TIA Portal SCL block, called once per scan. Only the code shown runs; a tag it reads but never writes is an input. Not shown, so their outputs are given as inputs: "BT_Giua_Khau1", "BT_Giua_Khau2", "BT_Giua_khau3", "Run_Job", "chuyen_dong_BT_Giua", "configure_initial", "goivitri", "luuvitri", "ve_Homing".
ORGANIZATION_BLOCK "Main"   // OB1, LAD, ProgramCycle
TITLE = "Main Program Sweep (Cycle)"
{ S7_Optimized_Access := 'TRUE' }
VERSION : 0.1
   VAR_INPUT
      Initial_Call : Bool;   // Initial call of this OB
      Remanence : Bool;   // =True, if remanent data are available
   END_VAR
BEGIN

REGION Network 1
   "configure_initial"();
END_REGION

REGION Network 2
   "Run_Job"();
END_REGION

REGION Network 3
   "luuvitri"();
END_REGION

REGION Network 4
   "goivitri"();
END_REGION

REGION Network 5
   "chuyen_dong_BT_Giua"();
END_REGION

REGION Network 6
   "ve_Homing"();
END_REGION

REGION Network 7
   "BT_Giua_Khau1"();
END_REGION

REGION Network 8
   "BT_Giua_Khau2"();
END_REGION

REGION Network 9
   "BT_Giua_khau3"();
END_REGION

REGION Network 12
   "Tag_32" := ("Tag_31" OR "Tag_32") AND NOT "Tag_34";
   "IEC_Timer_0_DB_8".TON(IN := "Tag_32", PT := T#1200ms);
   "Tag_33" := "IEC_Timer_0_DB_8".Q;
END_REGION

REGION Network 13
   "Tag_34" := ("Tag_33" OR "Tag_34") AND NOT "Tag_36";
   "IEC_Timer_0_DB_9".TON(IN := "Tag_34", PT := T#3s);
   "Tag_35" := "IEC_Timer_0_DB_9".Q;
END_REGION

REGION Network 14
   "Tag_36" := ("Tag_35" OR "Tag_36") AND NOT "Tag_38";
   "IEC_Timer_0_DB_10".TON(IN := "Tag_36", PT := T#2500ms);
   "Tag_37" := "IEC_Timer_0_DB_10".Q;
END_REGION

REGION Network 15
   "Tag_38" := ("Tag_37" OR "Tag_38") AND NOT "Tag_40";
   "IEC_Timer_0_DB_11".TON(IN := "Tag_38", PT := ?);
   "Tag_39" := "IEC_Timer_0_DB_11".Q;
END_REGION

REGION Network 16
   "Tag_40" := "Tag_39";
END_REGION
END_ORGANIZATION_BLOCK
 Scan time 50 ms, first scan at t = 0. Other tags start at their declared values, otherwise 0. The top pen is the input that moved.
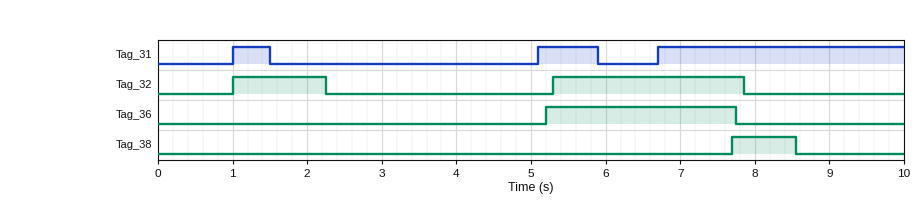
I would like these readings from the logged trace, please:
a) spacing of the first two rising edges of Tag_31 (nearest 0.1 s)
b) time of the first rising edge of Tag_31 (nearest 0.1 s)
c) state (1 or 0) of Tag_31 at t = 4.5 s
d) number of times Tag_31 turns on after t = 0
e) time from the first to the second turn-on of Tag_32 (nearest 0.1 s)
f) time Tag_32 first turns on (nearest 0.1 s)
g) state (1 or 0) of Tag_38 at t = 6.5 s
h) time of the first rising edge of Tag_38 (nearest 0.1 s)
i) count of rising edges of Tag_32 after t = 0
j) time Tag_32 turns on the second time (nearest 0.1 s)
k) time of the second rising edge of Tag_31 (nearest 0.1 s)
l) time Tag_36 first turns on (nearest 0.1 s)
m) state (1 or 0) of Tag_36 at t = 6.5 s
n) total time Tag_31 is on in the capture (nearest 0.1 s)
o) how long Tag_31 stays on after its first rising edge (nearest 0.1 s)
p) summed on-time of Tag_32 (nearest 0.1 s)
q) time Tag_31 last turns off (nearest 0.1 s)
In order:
4.1 s
1.0 s
0
3
4.3 s
1.0 s
0
7.7 s
2
5.3 s
5.1 s
5.2 s
1
4.6 s
0.5 s
3.8 s
5.9 s
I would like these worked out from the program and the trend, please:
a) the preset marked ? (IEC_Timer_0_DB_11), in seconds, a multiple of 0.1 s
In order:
0.8 s
